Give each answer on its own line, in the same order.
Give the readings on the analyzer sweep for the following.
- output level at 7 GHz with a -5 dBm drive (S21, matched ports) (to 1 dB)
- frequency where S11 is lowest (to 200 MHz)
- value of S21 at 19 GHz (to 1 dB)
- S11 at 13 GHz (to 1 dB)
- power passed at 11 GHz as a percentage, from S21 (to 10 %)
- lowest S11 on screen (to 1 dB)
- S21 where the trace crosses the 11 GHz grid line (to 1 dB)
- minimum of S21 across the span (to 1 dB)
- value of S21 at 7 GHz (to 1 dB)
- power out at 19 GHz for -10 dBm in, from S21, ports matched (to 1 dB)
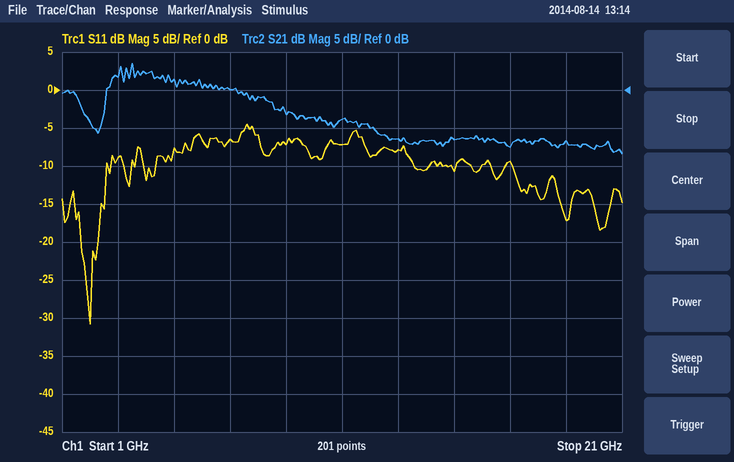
-5 dBm
2.0 GHz
-7 dB
-8 dB
40 %
-31 dB
-4 dB
-8 dB
0 dB
-17 dBm
